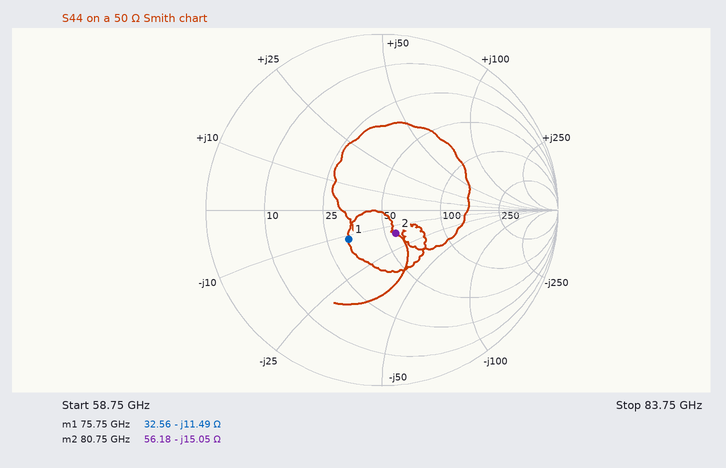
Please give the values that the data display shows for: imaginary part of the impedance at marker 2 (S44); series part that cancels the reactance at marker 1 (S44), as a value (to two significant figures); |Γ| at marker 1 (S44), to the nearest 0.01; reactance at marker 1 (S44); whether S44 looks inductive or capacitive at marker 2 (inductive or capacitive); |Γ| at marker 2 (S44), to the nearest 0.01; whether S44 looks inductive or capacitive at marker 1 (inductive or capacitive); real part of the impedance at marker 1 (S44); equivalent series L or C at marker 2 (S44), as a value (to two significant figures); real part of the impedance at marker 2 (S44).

-15.05 Ω
24 pH
0.25
-11.49 Ω
capacitive
0.15
capacitive
32.56 Ω
130 fF
56.18 Ω
